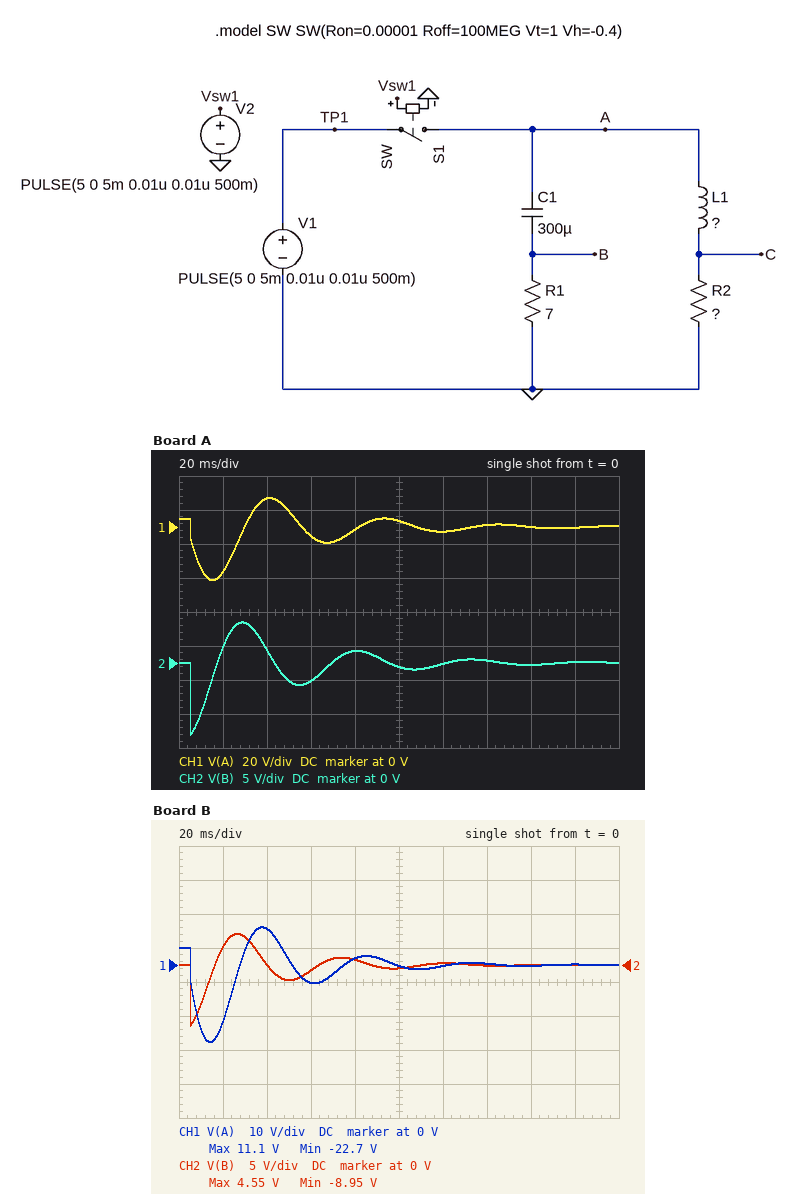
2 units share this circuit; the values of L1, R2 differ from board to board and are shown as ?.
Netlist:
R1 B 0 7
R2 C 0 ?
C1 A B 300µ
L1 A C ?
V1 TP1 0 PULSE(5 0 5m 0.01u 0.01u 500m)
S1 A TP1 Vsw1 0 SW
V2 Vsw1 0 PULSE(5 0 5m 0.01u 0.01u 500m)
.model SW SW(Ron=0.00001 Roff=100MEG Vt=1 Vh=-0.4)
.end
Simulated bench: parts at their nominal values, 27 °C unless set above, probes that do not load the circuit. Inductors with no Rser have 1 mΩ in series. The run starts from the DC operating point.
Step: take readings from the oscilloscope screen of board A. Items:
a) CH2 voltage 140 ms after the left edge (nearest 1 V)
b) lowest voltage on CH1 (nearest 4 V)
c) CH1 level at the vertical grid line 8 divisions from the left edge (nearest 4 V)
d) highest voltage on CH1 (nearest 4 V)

0 V
-32 V
0 V
16 V
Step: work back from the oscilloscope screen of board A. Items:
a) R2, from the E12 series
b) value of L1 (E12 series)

3.3 Ω
220 mH
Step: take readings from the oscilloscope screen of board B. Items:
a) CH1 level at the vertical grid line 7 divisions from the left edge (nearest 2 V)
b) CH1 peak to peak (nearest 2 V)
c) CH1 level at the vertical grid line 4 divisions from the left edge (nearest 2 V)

0 V
34 V
2 V
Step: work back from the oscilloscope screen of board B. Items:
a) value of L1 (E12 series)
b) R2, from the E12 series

180 mH
3.9 Ω
